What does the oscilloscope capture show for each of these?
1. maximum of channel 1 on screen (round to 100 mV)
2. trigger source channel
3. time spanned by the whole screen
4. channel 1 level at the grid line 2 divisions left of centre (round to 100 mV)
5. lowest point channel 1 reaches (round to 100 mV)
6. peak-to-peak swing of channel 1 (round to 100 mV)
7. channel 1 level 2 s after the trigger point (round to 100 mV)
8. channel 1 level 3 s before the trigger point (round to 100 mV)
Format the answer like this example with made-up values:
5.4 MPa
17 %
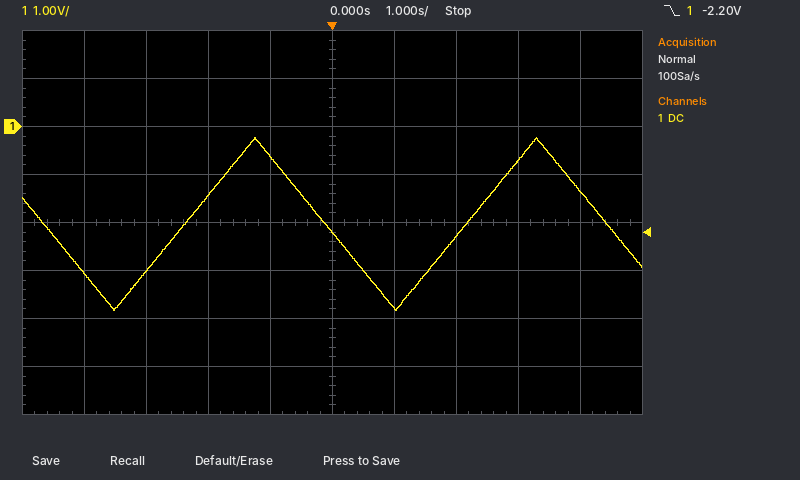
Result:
-200 mV
channel 1
10 s
-1.4 V
-3.8 V
3.6 V
-2.3 V
-3.0 V
